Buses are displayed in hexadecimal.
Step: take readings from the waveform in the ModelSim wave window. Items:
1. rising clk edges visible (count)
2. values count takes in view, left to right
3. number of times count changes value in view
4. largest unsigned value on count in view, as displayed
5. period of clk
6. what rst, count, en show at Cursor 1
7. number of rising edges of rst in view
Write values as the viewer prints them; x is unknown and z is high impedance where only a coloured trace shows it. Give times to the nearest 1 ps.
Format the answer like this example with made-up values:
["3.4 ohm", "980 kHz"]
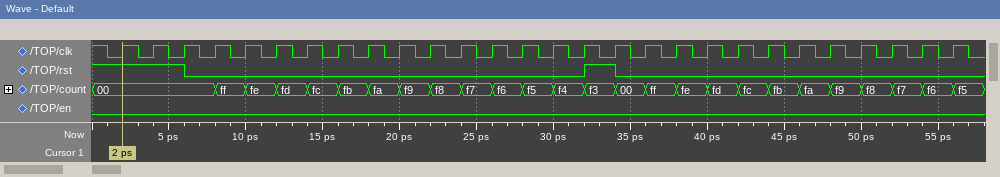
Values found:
["28", "00, ff, fe, fd, fc, fb, fa, f9, f8, f7, f6, f5, f4, f3, 00, ff, fe, fd, fc, fb, fa, f9, f8, f7, f6, f5", "25", "ff", "2 ps", "rst=1, count=00, en=0", "1"]
